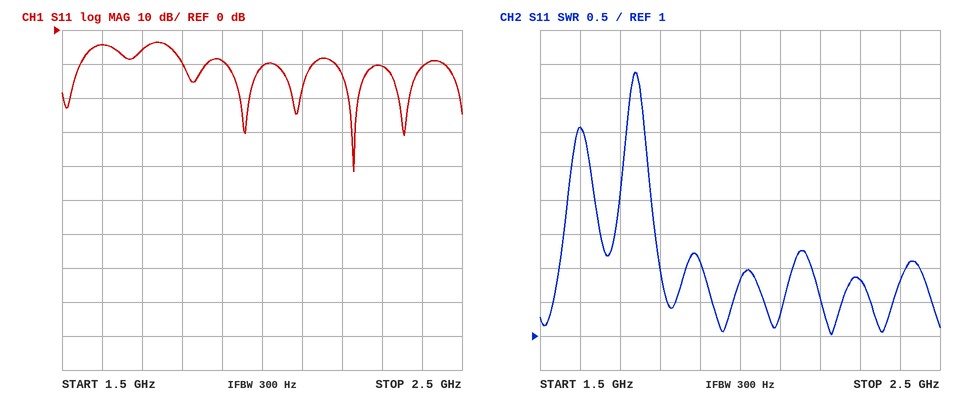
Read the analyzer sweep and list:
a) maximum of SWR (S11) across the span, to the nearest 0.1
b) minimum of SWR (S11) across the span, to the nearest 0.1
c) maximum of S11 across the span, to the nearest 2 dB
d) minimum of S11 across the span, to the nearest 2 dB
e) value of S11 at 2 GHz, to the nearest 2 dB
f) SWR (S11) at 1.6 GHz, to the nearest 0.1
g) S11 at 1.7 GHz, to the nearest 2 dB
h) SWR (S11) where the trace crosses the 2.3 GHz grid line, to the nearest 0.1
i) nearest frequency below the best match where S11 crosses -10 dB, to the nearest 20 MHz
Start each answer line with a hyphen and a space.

- 4.9
- 1.0
- -4 dB
- -42 dB
- -10 dB
- 4.1
- -6 dB
- 1.8
- 2.18 GHz
